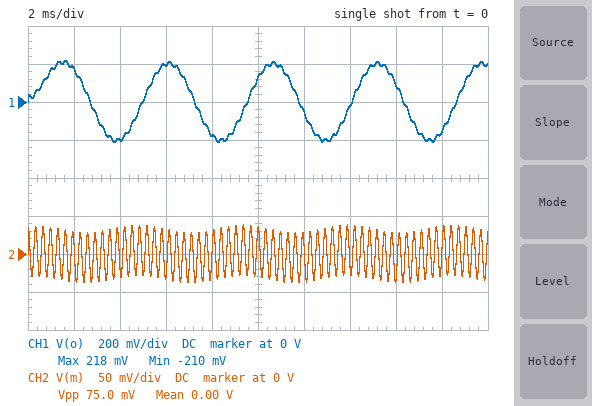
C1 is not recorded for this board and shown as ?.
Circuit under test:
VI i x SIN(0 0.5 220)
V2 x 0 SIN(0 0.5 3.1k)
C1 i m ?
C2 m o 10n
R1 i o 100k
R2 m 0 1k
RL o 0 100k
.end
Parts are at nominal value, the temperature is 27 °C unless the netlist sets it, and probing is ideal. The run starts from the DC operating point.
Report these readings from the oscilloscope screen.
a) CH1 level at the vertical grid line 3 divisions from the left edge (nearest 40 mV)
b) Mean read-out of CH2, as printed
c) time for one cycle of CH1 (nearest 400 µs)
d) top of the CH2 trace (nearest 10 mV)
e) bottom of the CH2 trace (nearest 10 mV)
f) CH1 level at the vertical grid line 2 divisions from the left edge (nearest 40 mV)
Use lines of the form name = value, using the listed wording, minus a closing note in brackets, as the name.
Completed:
CH1 level at the vertical grid line 3 divisions from the left edge = 200 mV
Mean read-out of CH2, as printed = 0.00 V
time for one cycle of CH1 = 4.4 ms
top of the CH2 trace = 40 mV
bottom of the CH2 trace = -40 mV
CH1 level at the vertical grid line 2 divisions from the left edge = -200 mV
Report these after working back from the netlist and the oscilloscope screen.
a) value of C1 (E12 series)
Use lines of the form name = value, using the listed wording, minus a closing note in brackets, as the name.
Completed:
value of C1 = 3.3 nF
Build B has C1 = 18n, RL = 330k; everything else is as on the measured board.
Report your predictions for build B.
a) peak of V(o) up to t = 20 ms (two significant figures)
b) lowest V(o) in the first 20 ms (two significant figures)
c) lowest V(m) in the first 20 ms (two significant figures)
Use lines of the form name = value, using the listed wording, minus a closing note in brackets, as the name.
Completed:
peak of V(o) up to t = 20 ms = 420 mV
lowest V(o) in the first 20 ms = -390 mV
lowest V(m) in the first 20 ms = -180 mV
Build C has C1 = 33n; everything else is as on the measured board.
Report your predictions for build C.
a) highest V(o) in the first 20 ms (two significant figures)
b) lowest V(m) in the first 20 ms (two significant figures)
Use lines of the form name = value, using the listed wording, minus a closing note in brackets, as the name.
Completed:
highest V(o) in the first 20 ms = 440 mV
lowest V(m) in the first 20 ms = -290 mV
